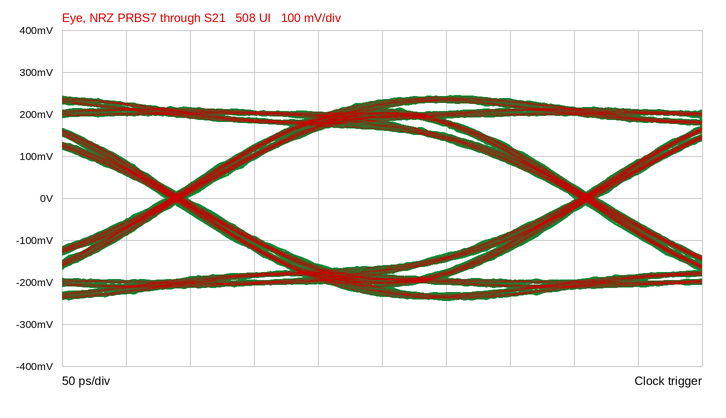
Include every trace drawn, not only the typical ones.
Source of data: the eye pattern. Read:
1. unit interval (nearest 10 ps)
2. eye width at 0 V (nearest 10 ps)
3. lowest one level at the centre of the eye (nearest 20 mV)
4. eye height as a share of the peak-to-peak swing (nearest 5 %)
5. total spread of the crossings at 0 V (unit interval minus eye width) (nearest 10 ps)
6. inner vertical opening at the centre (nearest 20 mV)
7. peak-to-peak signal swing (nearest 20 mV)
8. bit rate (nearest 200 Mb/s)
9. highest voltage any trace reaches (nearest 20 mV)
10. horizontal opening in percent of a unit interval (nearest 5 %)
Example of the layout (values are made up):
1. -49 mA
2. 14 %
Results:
1. 320 ps
2. 300 ps
3. 160 mV
4. 65 %
5. 20 ps
6. 320 mV
7. 480 mV
8. 3.2 Gb/s
9. 240 mV
10. 95 %
